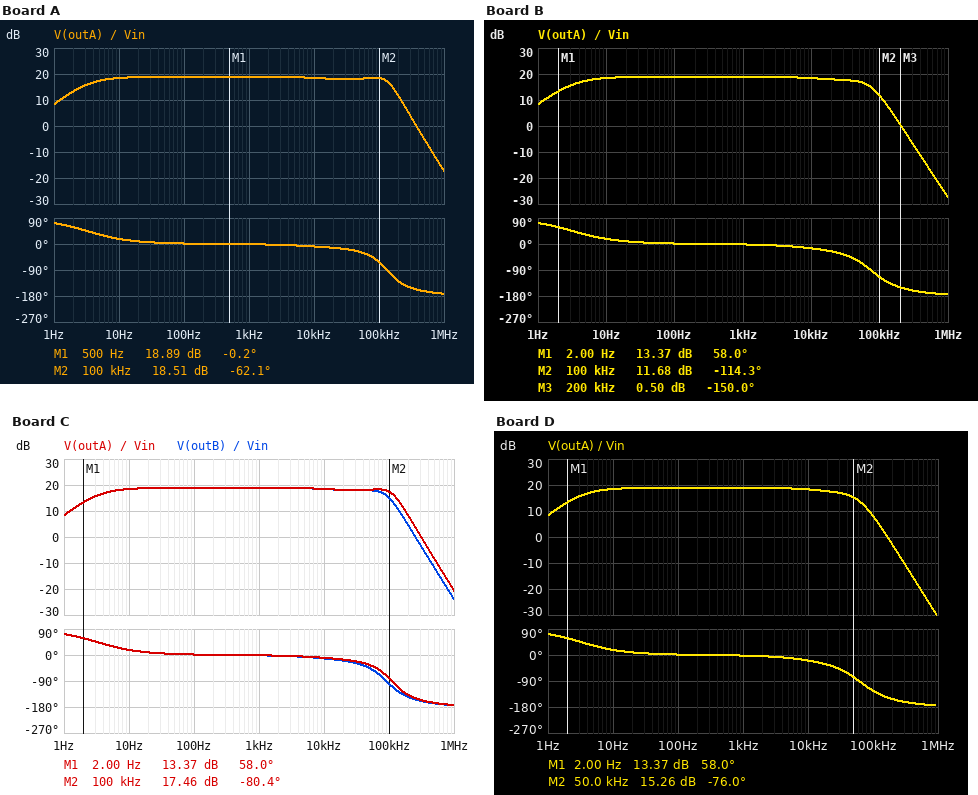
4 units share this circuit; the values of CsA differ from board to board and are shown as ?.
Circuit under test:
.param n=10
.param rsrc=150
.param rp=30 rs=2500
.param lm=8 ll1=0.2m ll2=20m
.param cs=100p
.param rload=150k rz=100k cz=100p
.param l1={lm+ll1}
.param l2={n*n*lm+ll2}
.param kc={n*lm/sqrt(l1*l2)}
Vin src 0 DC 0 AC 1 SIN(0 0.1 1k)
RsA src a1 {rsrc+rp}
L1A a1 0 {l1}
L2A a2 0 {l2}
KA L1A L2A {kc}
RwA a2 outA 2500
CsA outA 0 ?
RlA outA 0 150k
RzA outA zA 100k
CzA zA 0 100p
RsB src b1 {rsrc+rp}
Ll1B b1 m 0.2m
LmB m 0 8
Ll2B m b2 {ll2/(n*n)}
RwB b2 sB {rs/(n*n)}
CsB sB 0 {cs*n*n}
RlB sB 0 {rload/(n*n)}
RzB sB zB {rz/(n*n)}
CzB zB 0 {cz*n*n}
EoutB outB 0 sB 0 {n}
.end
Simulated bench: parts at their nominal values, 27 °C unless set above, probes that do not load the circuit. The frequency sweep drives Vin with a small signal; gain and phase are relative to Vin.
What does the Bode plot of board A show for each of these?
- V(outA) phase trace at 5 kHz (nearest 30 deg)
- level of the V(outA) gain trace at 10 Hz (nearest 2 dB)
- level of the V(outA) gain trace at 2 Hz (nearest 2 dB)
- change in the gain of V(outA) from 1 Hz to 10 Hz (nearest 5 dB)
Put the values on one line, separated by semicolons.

0 deg; 18 dB; 14 dB; 10 dB
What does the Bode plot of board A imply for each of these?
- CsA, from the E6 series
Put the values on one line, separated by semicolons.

47 pF
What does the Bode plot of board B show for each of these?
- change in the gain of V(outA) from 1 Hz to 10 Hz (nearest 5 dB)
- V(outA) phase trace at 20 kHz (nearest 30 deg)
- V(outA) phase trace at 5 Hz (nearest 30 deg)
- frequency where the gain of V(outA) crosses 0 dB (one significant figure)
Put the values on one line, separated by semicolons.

10 dB; -30 deg; 30 deg; 200 kHz
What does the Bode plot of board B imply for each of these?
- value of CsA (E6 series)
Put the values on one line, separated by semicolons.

150 pF
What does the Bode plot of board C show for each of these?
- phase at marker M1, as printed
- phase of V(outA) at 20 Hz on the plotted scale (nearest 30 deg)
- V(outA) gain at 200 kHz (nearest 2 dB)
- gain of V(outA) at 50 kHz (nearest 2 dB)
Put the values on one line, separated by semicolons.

58.0 deg; 0 deg; 8 dB; 18 dB
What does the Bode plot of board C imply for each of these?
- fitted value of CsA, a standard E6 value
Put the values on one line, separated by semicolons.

68 pF
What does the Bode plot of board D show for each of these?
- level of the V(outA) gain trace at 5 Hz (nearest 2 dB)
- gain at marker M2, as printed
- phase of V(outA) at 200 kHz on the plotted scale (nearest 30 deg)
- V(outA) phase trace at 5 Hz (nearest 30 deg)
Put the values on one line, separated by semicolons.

18 dB; 15.26 dB; -150 deg; 30 deg
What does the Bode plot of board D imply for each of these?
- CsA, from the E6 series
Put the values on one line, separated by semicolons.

220 pF
